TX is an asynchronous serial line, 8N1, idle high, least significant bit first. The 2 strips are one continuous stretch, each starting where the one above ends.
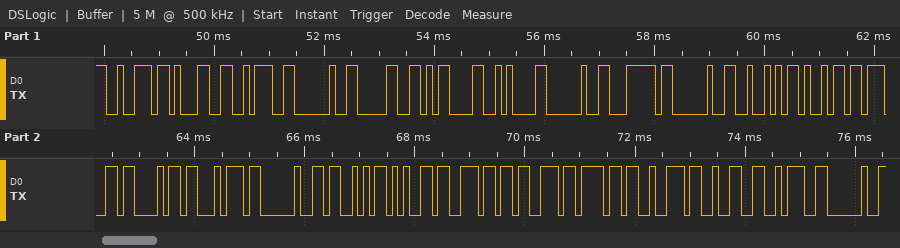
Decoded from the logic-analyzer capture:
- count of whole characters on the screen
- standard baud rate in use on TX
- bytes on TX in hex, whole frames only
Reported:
25
9600 baud
72 31 3A 20 30 0D 0A 20 7C 20 52 69 67 68 74 20 53 65 6E 73 6F 72 32 3A 20
